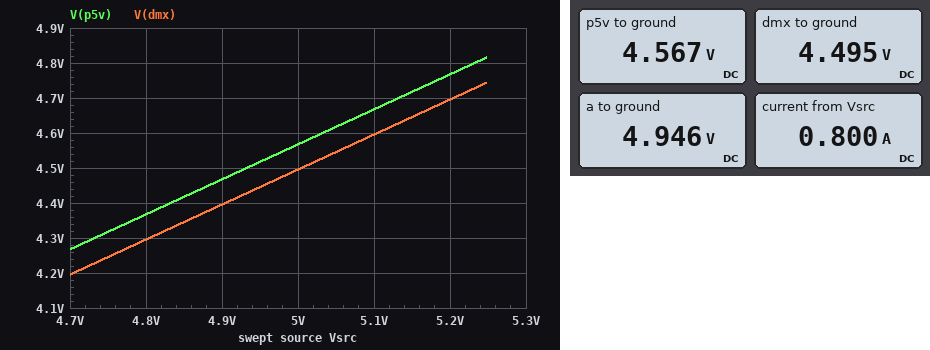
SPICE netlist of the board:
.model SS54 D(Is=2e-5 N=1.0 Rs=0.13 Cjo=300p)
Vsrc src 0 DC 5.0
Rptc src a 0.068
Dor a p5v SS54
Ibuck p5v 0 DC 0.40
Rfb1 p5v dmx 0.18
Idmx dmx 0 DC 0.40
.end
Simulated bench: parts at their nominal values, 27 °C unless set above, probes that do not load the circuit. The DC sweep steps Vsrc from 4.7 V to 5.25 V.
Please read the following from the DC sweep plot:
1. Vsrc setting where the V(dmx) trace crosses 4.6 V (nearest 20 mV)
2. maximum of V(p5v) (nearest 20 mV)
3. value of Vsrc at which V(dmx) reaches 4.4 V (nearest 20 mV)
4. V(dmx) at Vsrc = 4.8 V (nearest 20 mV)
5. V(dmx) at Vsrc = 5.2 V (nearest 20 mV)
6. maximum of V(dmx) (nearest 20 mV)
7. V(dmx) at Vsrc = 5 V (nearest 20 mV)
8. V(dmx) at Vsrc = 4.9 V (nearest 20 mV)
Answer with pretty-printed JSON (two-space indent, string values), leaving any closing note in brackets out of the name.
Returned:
{
  "Vsrc setting where the V(dmx) trace crosses 4.6 V": "5.10 V",
  "maximum of V(p5v)": "4.82 V",
  "value of Vsrc at which V(dmx) reaches 4.4 V": "4.90 V",
  "V(dmx) at Vsrc = 4.8 V": "4.30 V",
  "V(dmx) at Vsrc = 5.2 V": "4.70 V",
  "maximum of V(dmx)": "4.74 V",
  "V(dmx) at Vsrc = 5 V": "4.50 V",
  "V(dmx) at Vsrc = 4.9 V": "4.40 V"
}
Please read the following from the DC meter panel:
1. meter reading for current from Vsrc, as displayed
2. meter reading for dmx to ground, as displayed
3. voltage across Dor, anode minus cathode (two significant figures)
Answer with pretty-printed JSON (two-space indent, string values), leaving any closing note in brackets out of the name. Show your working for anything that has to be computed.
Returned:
{
  "meter reading for current from Vsrc, as displayed": "0.800 A",
  "meter reading for dmx to ground, as displayed": "4.495 V",
  "voltage across Dor, anode minus cathode": "4.946 V - 4.567 V = 380 mV"
}
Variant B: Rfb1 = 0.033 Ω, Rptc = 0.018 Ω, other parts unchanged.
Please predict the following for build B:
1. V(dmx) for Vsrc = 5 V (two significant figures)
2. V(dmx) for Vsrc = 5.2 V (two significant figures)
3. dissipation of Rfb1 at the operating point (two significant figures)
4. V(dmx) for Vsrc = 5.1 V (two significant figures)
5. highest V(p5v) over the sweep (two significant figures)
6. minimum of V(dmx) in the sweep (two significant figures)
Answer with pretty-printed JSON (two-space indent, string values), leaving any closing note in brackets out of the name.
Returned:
{
  "V(dmx) for Vsrc = 5 V": "4.6 V",
  "V(dmx) for Vsrc = 5.2 V": "4.8 V",
  "dissipation of Rfb1 at the operating point": "5.3 mW",
  "V(dmx) for Vsrc = 5.1 V": "4.7 V",
  "highest V(p5v) over the sweep": "4.9 V",
  "minimum of V(dmx) in the sweep": "4.3 V"
}
